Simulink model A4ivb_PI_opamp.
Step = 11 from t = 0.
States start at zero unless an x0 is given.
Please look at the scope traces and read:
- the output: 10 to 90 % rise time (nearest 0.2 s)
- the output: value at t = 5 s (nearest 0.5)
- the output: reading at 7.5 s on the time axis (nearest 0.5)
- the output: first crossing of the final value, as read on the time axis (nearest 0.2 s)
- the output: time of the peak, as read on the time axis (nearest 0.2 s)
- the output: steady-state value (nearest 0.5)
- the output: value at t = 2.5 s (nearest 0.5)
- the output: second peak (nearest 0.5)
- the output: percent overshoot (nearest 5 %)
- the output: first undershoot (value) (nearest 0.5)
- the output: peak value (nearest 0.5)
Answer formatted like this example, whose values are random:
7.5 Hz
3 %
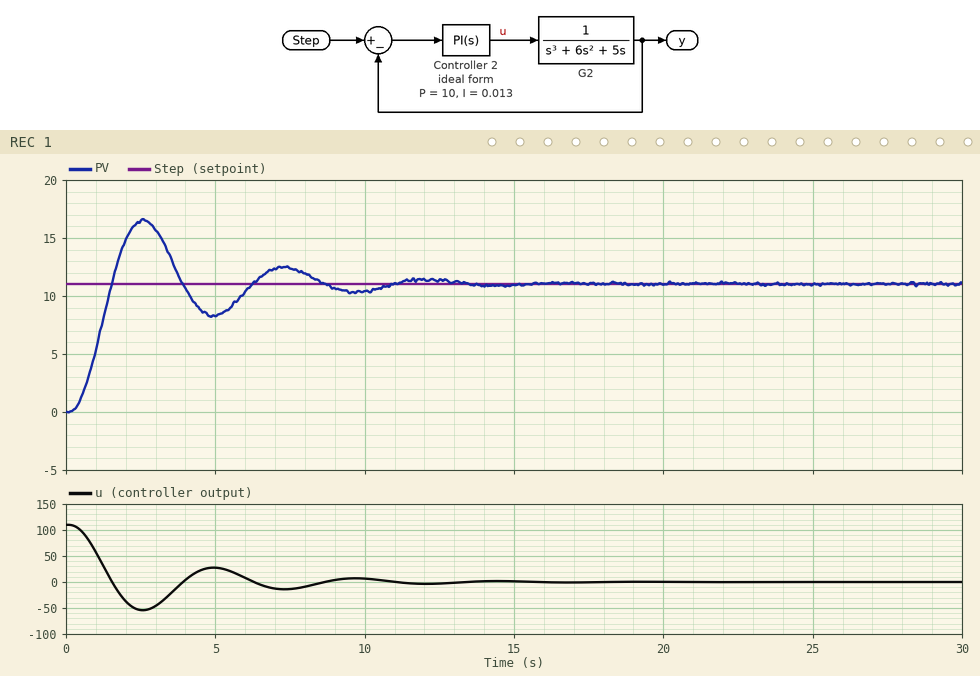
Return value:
1.0 s
8.5
12.5
1.6 s
2.6 s
11.0
16.5
12.5
50 %
8.5
16.5
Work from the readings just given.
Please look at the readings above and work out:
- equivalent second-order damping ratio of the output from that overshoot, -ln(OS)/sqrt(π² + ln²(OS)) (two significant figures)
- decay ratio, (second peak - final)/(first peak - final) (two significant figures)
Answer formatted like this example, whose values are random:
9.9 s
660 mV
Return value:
0.22
0.27
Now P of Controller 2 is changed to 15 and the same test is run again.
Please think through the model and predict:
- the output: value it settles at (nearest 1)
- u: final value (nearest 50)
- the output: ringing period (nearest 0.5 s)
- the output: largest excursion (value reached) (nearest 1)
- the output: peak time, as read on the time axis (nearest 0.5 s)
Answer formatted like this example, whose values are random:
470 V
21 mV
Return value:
11
0
4.0 s
18
2.0 s
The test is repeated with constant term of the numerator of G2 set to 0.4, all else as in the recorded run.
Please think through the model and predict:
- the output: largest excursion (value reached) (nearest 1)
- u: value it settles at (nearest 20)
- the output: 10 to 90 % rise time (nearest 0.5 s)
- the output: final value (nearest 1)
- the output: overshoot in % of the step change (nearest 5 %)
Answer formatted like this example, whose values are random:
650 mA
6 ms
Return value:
13
0
2.0 s
11
20 %
